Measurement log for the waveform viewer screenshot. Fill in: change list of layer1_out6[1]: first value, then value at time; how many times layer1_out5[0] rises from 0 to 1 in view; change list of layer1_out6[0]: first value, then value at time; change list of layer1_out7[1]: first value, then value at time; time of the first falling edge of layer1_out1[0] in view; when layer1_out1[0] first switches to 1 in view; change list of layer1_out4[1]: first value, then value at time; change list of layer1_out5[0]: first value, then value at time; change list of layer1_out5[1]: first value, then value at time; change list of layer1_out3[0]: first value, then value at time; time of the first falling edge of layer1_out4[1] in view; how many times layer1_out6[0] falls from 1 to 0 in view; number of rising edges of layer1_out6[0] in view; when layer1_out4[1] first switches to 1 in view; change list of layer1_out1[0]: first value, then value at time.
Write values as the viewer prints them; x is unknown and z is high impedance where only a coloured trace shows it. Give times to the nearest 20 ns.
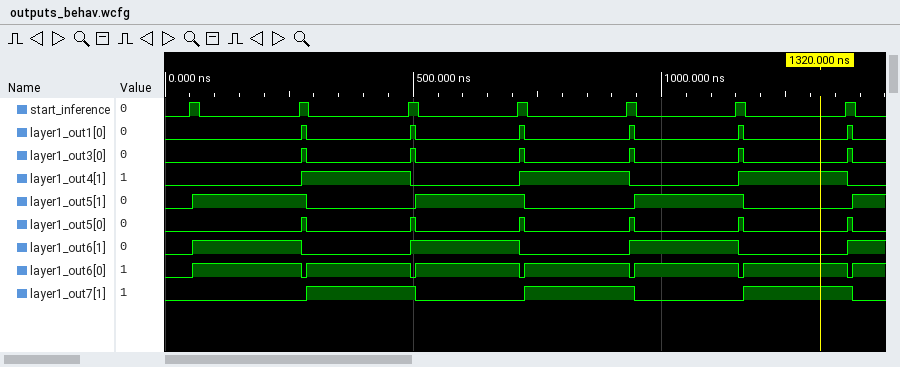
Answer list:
0, 1 at 60 ns, 0 at 280 ns, 1 at 500 ns, 0 at 720 ns, 1 at 940 ns, 0 at 1160 ns, 1 at 1380 ns
6
0, 1 at 60 ns, 0 at 280 ns, 1 at 280 ns, 0 at 500 ns, 1 at 500 ns, 0 at 720 ns, 1 at 720 ns, 0 at 940 ns, 1 at 940 ns, 0 at 1160 ns, 1 at 1160 ns, 0 at 1380 ns, 1 at 1380 ns
0, 1 at 280 ns, 0 at 500 ns, 1 at 720 ns, 0 at 940 ns, 1 at 1160 ns, 0 at 1380 ns
280 ns
280 ns
0, 1 at 280 ns, 0 at 500 ns, 1 at 720 ns, 0 at 940 ns, 1 at 1160 ns, 0 at 1380 ns
0, 1 at 280 ns, 0 at 280 ns, 1 at 500 ns, 0 at 500 ns, 1 at 720 ns, 0 at 720 ns, 1 at 940 ns, 0 at 940 ns, 1 at 1160 ns, 0 at 1160 ns, 1 at 1380 ns, 0 at 1380 ns
0, 1 at 60 ns, 0 at 280 ns, 1 at 500 ns, 0 at 720 ns, 1 at 940 ns, 0 at 1160 ns, 1 at 1380 ns
0, 1 at 280 ns, 0 at 280 ns, 1 at 500 ns, 0 at 500 ns, 1 at 720 ns, 0 at 720 ns, 1 at 940 ns, 0 at 940 ns, 1 at 1160 ns, 0 at 1160 ns, 1 at 1380 ns, 0 at 1380 ns
500 ns
6
7
280 ns
0, 1 at 280 ns, 0 at 280 ns, 1 at 500 ns, 0 at 500 ns, 1 at 720 ns, 0 at 720 ns, 1 at 940 ns, 0 at 940 ns, 1 at 1160 ns, 0 at 1160 ns, 1 at 1380 ns, 0 at 1380 ns
